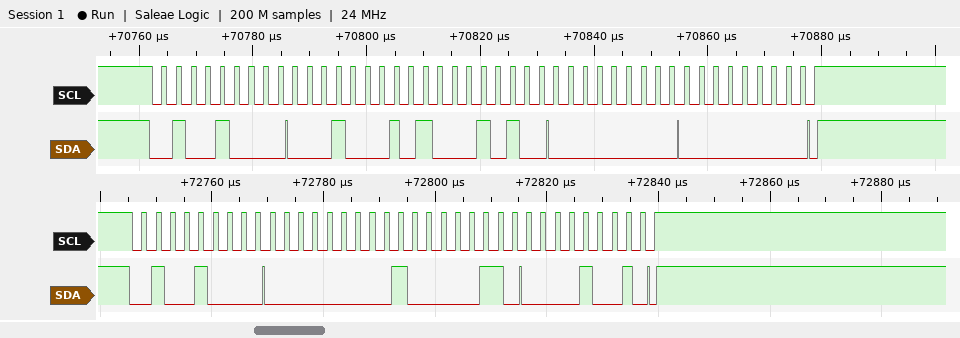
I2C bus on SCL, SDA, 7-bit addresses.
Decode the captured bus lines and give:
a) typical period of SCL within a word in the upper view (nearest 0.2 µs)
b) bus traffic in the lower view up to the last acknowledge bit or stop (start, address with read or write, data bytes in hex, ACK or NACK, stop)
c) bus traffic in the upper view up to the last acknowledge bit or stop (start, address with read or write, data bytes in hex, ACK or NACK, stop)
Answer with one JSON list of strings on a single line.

["2.6 µs", "start, address 24 write ACK, 00 ACK, 83 ACK, 09 ACK, stop", "start, address 24 write ACK, 11 ACK, 8A ACK, 00 ACK, 00 ACK, stop"]
